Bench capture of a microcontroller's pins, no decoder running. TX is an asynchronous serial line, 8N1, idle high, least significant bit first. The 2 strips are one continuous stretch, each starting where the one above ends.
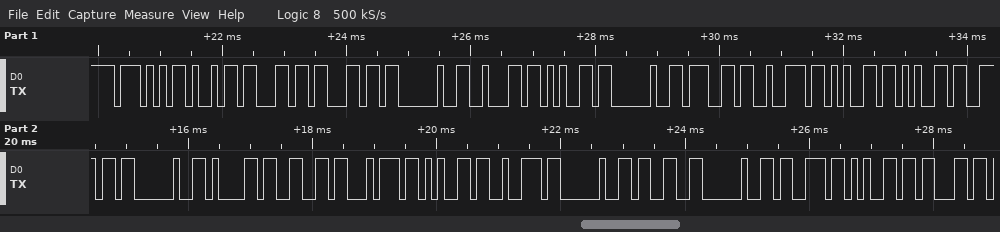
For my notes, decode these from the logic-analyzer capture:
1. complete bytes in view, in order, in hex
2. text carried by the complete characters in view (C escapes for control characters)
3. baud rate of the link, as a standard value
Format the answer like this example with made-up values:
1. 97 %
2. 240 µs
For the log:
1. 57 69 6C 6C 20 62 65 20 67 72 65 65 6E 20 61 66 74 65 72 20 33 20 73 65 63
2. "Will be green after 3 sec"
3. 9600 baud
